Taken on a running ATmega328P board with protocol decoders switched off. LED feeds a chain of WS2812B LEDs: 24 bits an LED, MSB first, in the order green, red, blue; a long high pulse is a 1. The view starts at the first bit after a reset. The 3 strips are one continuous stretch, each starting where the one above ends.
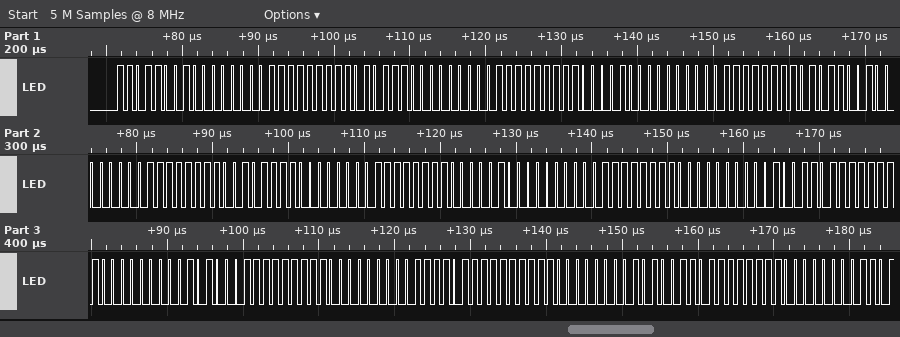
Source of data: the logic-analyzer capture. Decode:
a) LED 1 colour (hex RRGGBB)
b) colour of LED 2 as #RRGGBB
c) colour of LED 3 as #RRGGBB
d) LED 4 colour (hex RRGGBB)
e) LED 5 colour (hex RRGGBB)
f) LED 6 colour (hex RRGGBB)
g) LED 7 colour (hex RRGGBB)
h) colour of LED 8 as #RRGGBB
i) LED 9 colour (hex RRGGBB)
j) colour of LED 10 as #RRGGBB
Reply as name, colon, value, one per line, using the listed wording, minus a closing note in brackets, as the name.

LED 1 colour: #00D9FF
colour of LED 2 as #RRGGBB: #00AEFF
colour of LED 3 as #RRGGBB: #0084FF
LED 4 colour: #0059FF
LED 5 colour: #002FFF
LED 6 colour: #0004FF
LED 7 colour: #2600FF
colour of LED 8 as #RRGGBB: #5100FF
LED 9 colour: #7B00FF
colour of LED 10 as #RRGGBB: #A600FF
